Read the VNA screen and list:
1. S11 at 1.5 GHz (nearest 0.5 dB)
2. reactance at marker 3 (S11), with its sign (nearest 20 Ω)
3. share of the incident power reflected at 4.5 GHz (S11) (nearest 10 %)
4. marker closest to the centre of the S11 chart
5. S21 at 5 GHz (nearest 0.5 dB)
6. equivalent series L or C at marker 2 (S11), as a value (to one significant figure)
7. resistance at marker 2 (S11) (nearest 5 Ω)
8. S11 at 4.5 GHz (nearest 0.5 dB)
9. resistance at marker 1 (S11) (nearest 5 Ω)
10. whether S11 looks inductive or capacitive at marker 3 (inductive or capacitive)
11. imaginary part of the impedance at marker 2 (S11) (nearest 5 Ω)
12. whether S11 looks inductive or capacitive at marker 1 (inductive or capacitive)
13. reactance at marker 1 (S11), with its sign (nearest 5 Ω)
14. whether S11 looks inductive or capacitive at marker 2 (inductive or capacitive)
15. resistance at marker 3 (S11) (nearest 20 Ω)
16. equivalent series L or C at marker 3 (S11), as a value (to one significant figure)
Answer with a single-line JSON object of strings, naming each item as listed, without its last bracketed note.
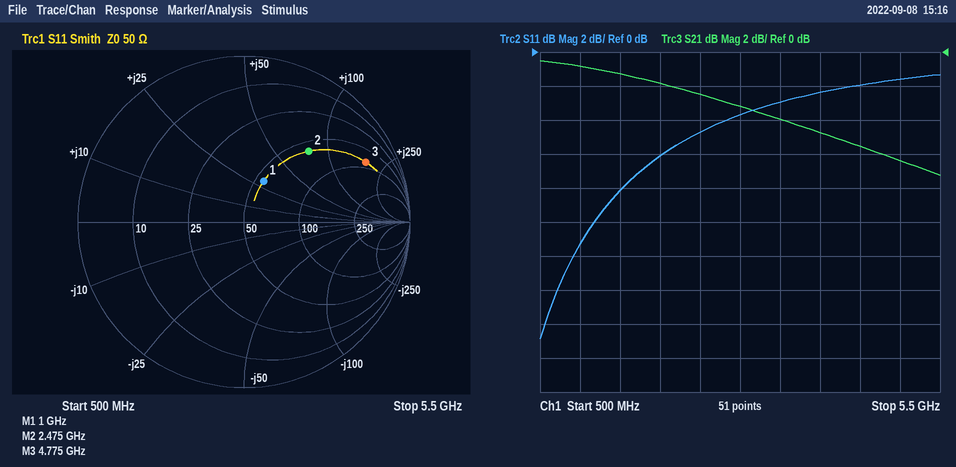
{"S11 at 1.5 GHz": "-8.0 dB", "reactance at marker 3 (S11), with its sign": "+180 Ω", "share of the incident power reflected at 4.5 GHz (S11)": "60 %", "marker closest to the centre of the S11 chart": "marker 1", "S21 at 5 GHz": "-6.5 dB", "equivalent series L or C at marker 2 (S11), as a value": "5 nH", "resistance at marker 2 (S11)": "60 Ω", "S11 at 4.5 GHz": "-2.0 dB", "resistance at marker 1 (S11)": "55 Ω", "whether S11 looks inductive or capacitive at marker 3": "inductive", "imaginary part of the impedance at marker 2 (S11)": "+75 Ω", "whether S11 looks inductive or capacitive at marker 1": "inductive", "reactance at marker 1 (S11), with its sign": "+30 Ω", "whether S11 looks inductive or capacitive at marker 2": "inductive", "resistance at marker 3 (S11)": "80 Ω", "equivalent series L or C at marker 3 (S11), as a value": "6 nH"}
